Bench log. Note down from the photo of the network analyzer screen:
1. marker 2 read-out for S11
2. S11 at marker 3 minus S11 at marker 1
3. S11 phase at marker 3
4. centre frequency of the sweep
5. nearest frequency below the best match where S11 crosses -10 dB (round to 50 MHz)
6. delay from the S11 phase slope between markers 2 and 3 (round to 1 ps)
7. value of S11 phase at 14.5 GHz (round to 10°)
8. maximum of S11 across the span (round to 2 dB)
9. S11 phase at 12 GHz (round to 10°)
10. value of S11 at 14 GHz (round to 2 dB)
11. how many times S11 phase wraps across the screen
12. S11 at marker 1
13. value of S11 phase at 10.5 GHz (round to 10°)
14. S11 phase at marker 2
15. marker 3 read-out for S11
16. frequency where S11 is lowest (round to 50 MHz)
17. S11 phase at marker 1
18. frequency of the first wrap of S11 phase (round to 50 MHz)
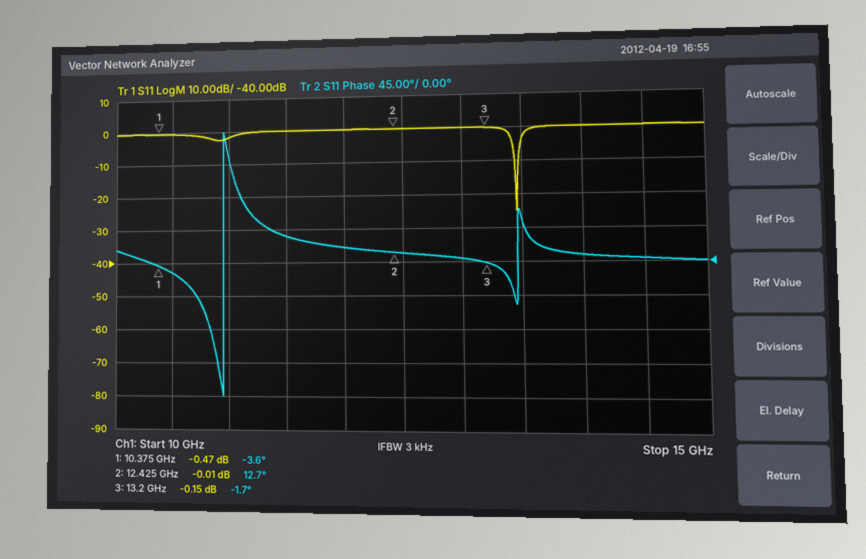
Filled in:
-0.01 dB
0.32 dB
-1.7°
12.5 GHz
13.45 GHz
52 ps
0°
0 dB
20°
0 dB
1
-0.47 dB
-10°
12.7°
-0.15 dB
13.45 GHz
-3.6°
10.95 GHz
